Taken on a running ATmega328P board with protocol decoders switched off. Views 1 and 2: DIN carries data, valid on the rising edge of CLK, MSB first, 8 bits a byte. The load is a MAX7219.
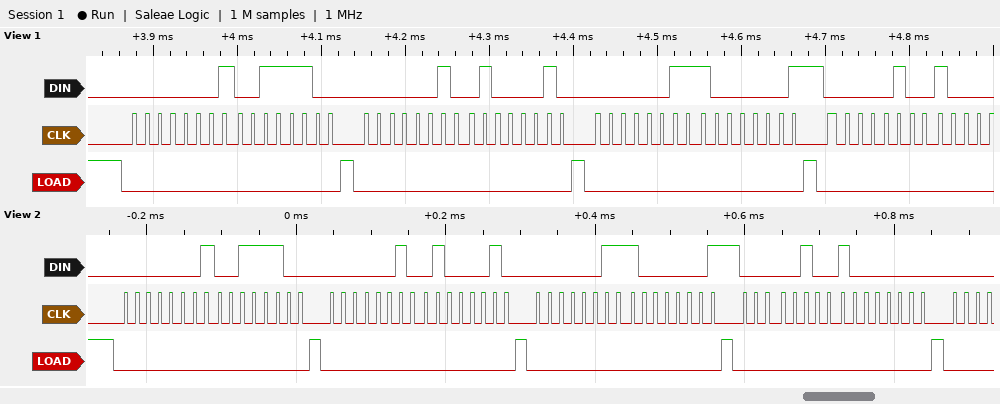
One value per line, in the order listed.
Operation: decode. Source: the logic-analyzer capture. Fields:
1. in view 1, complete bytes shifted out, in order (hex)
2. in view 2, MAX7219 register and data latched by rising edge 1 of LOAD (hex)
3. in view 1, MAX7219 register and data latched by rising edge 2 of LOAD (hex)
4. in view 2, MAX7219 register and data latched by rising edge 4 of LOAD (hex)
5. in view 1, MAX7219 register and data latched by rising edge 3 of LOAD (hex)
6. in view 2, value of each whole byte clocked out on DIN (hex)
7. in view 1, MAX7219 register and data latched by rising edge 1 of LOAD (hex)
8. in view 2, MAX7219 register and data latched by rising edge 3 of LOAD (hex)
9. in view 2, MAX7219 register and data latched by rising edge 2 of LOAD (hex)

0x01 0x3C 0x02 0x42 0x03 0x81 0x04
register 0x1, data 0x3C
register 0x2, data 0x42
register 0x4, data 0x80
register 0x3, data 0x81
0x01 0x3C 0x02 0x42 0x03 0x81 0x04 0x80
register 0x1, data 0x3C
register 0x3, data 0x81
register 0x2, data 0x42
